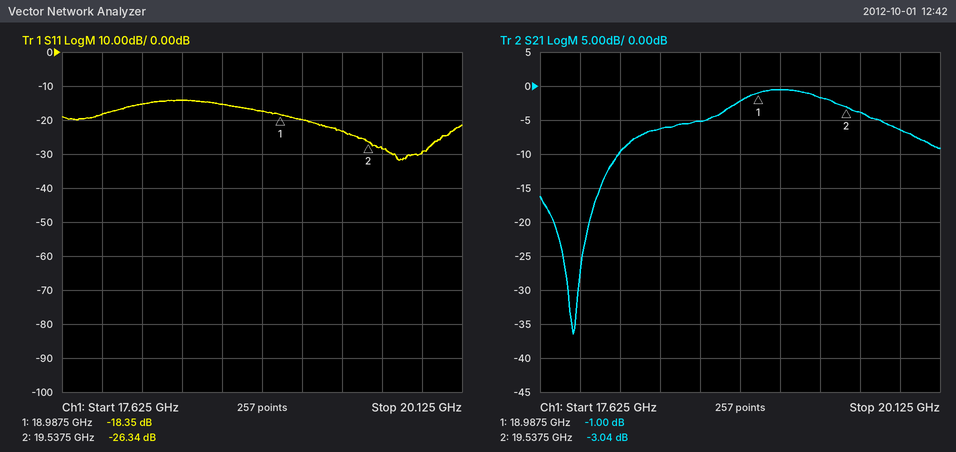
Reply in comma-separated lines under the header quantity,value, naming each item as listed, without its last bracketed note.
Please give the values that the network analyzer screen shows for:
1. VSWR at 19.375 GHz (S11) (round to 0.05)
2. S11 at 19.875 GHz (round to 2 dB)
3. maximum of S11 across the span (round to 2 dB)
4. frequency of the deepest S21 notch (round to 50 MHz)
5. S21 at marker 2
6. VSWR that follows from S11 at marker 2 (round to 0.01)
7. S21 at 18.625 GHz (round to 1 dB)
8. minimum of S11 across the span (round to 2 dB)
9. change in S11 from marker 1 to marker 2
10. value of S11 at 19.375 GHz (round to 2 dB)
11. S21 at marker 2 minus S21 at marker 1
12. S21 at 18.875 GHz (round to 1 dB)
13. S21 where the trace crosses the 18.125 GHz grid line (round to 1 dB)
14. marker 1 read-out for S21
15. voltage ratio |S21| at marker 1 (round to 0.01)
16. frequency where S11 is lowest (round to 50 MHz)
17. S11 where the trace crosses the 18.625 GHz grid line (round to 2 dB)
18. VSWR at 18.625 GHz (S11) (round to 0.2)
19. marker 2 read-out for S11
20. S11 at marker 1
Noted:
quantity,value
VSWR at 19.375 GHz (S11),1.15
S11 at 19.875 GHz,-30 dB
maximum of S11 across the span,-14 dB
frequency of the deepest S21 notch,17.85 GHz
S21 at marker 2,-3.04 dB
VSWR that follows from S11 at marker 2,1.10
S21 at 18.625 GHz,-5 dB
minimum of S11 across the span,-32 dB
change in S11 from marker 1 to marker 2,-7.99 dB
value of S11 at 19.375 GHz,-24 dB
S21 at marker 2 minus S21 at marker 1,-2.04 dB
S21 at 18.875 GHz,-2 dB
S21 where the trace crosses the 18.125 GHz grid line,-10 dB
marker 1 read-out for S21,-1.00 dB
voltage ratio |S21| at marker 1,0.89
frequency where S11 is lowest,19.75 GHz
S11 where the trace crosses the 18.625 GHz grid line,-16 dB
VSWR at 18.625 GHz (S11),1.4
marker 2 read-out for S11,-26.34 dB
S11 at marker 1,-18.35 dB
